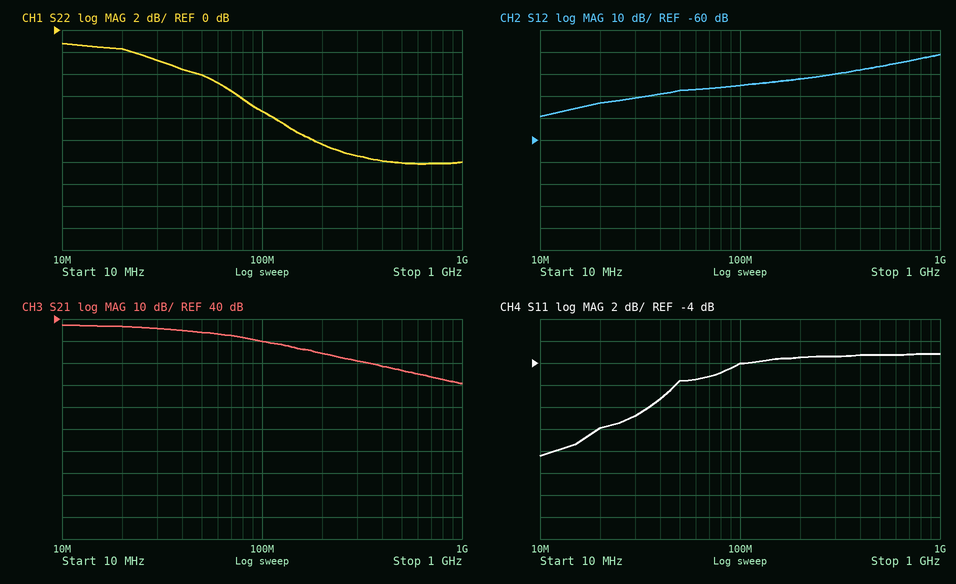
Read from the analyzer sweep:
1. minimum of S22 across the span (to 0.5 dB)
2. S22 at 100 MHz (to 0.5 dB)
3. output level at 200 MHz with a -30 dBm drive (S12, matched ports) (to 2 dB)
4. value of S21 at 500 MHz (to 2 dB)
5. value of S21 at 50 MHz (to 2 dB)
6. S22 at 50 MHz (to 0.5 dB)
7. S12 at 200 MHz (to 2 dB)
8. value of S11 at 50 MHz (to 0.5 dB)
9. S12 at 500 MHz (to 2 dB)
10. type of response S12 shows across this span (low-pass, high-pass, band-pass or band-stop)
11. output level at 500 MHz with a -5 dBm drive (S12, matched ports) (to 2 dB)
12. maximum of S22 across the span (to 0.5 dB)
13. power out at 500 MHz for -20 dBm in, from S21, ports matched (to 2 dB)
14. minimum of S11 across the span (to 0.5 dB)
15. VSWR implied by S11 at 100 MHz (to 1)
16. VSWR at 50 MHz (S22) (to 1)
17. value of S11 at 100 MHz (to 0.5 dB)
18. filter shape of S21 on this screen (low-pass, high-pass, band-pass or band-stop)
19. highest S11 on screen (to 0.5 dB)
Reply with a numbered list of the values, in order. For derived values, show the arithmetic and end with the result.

1. -12.0 dB
2. -7.5 dB
3. -30 dBm + (-32 dB) = -62 dBm
4. 16 dB
5. 34 dB
6. -4.0 dB
7. -32 dB
8. -5.5 dB
9. -26 dB
10. high-pass
11. -5 dBm + (-26 dB) = -32 dBm
12. -1.0 dB
13. -20 dBm + (16 dB) = -4 dBm
14. -12.5 dB
15. |Γ| = 10^(-4/20) = 0.6310; VSWR = (1 + 0.6310)/(1 − 0.6310) ≈ 4
16. |Γ| = 10^(-4/20) = 0.6310; VSWR = (1 + 0.6310)/(1 − 0.6310) ≈ 4
17. -4.0 dB
18. low-pass
19. -3.0 dB
